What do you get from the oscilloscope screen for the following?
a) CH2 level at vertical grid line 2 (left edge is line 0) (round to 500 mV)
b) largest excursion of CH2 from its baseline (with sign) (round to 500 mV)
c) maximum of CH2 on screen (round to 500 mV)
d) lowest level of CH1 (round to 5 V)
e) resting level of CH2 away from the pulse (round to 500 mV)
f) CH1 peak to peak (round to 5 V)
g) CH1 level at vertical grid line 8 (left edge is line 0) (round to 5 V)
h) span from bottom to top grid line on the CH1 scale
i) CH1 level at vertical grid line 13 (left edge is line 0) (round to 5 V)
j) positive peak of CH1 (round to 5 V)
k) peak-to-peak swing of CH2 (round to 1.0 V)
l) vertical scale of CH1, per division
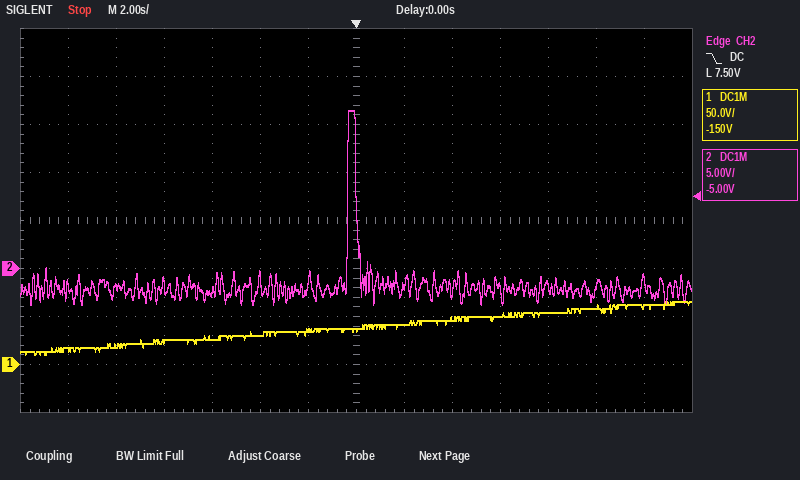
-2.0 V
+18.5 V
16.5 V
10 V
-2.0 V
55 V
40 V
400 V
60 V
65 V
20.0 V
50 V
